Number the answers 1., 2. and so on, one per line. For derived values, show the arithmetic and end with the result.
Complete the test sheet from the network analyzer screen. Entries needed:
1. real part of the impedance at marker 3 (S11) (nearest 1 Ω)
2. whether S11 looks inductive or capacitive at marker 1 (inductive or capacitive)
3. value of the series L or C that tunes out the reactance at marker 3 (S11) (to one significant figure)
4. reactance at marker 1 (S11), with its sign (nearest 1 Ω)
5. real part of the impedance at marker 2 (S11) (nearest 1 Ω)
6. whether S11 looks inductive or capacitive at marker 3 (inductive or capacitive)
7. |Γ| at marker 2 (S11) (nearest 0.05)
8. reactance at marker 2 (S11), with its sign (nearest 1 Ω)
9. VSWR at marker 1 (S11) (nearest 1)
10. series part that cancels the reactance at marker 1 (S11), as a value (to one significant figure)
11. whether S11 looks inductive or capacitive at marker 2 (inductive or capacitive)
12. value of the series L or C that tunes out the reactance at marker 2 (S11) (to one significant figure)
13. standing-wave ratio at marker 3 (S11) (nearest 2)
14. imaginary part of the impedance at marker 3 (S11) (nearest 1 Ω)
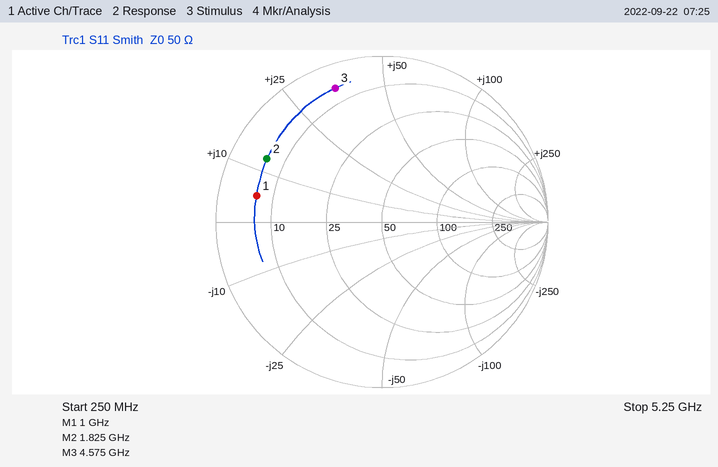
1. 6 Ω
2. inductive
3. C = 1/(2π × 4.575 GHz × 35 Ω) ≈ 1.0 pF
4. +5 Ω
5. 6 Ω
6. inductive
7. 0.80
8. +13 Ω
9. 8
10. C = 1/(2π × 1 GHz × 5 Ω) ≈ 31.8 pF, so 30 pF to one significant figure
11. inductive
12. C = 1/(2π × 1.825 GHz × 13 Ω) ≈ 7 pF
13. 12
14. +35 Ω
